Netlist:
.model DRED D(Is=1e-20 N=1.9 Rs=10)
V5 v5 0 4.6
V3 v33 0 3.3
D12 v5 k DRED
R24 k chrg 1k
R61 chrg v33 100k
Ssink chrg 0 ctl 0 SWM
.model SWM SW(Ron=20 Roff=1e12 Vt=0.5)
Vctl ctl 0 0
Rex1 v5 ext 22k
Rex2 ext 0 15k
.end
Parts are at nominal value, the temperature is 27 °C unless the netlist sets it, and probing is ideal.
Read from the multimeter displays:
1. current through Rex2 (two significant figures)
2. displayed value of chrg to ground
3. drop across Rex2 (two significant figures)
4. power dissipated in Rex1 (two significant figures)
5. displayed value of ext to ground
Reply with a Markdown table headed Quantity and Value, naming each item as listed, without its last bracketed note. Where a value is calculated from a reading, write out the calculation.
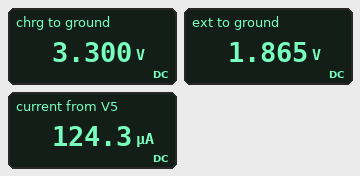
| Quantity | Value |
|---|---|
| current through Rex2 | (1.865 V) / 15 kΩ = 120 µA |
| displayed value of chrg to ground | 3.300 V |
| drop across Rex2 | 1.865 V = 1.9 V |
| power dissipated in Rex1 | (4.6 V - 1.865 V)^2 / 22 kΩ = 340 µW |
| displayed value of ext to ground | 1.865 V |
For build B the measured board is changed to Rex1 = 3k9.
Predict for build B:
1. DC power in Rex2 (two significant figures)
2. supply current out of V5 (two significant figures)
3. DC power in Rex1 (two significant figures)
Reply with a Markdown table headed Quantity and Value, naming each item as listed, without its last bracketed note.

| Quantity | Value |
|---|---|
| DC power in Rex2 | 890 µW |
| supply current out of V5 | 240 µA |
| DC power in Rex1 | 230 µW |
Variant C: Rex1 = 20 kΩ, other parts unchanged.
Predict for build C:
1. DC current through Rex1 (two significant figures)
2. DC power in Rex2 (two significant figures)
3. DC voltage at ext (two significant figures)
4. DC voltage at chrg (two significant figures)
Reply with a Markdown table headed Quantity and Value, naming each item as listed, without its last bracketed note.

| Quantity | Value |
|---|---|
| DC current through Rex1 | 130 µA |
| DC power in Rex2 | 260 µW |
| DC voltage at ext | 2.0 V |
| DC voltage at chrg | 3.3 V |
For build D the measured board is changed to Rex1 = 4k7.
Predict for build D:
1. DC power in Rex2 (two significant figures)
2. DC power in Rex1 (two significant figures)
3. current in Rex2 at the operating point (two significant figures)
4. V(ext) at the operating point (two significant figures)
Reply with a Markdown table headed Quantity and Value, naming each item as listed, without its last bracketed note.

| Quantity | Value |
|---|---|
| DC power in Rex2 | 820 µW |
| DC power in Rex1 | 260 µW |
| current in Rex2 at the operating point | 230 µA |
| V(ext) at the operating point | 3.5 V |
